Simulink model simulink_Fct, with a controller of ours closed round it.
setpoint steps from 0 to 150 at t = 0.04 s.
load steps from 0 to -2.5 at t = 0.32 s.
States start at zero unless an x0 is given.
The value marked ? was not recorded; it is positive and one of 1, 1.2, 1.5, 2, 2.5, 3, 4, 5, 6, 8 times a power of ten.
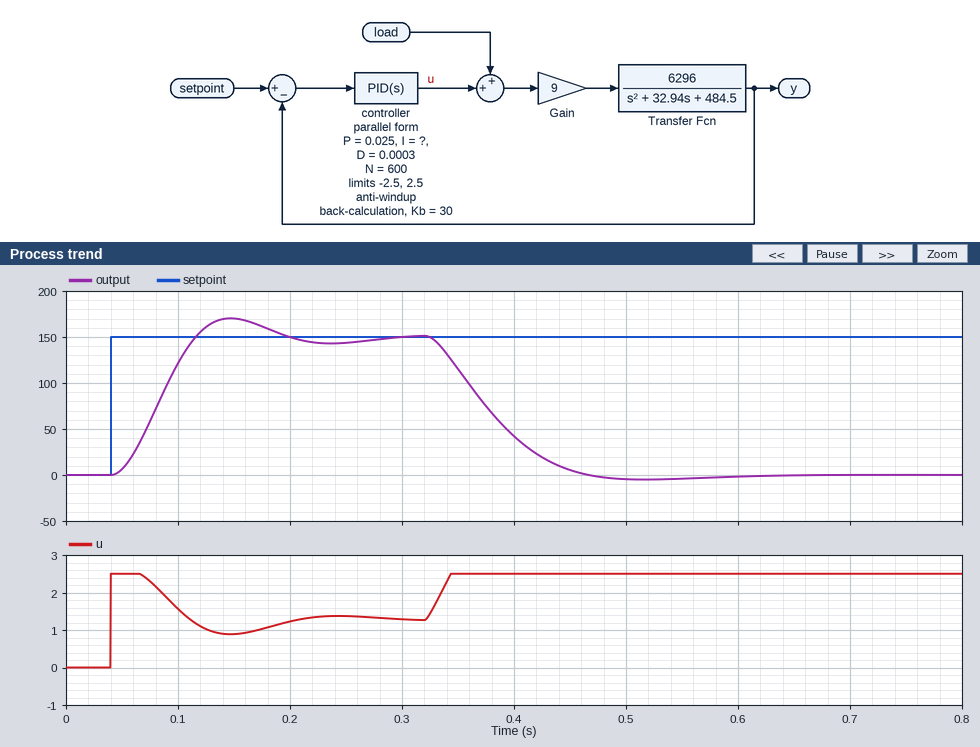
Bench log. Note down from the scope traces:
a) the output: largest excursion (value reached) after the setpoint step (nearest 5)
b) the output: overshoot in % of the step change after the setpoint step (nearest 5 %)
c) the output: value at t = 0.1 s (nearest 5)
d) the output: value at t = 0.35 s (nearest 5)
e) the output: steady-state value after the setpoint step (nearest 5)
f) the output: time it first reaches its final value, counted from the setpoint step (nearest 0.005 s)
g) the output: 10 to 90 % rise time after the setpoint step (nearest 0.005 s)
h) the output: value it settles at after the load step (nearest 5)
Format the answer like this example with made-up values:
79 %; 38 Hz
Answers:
170; 15 %; 120; 115; 150; 0.075 s; 0.050 s; 0
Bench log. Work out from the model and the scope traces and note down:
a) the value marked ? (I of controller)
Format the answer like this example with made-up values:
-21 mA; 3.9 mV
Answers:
0.5
